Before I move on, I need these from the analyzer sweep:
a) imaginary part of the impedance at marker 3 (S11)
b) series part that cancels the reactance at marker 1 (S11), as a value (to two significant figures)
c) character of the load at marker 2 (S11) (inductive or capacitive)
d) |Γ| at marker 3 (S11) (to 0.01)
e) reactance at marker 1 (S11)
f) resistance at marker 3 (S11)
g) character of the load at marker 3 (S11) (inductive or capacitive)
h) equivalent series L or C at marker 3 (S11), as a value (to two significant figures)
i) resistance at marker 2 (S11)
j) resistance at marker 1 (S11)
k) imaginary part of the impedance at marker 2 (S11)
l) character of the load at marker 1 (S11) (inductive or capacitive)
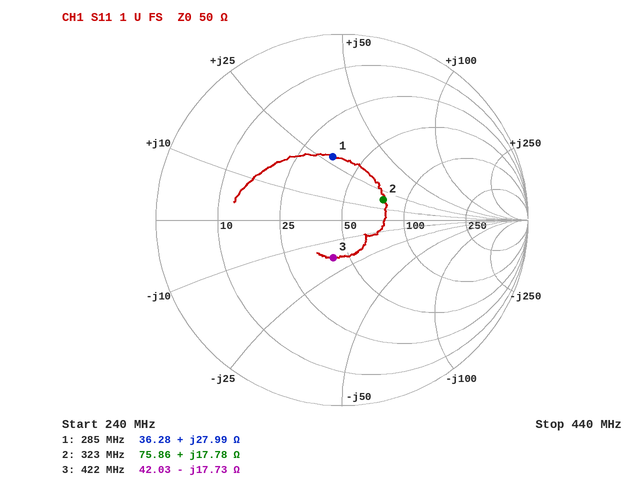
-17.73 Ω
20 pF
inductive
0.21
+27.99 Ω
42.03 Ω
capacitive
21 pF
75.86 Ω
36.28 Ω
+17.78 Ω
inductive
